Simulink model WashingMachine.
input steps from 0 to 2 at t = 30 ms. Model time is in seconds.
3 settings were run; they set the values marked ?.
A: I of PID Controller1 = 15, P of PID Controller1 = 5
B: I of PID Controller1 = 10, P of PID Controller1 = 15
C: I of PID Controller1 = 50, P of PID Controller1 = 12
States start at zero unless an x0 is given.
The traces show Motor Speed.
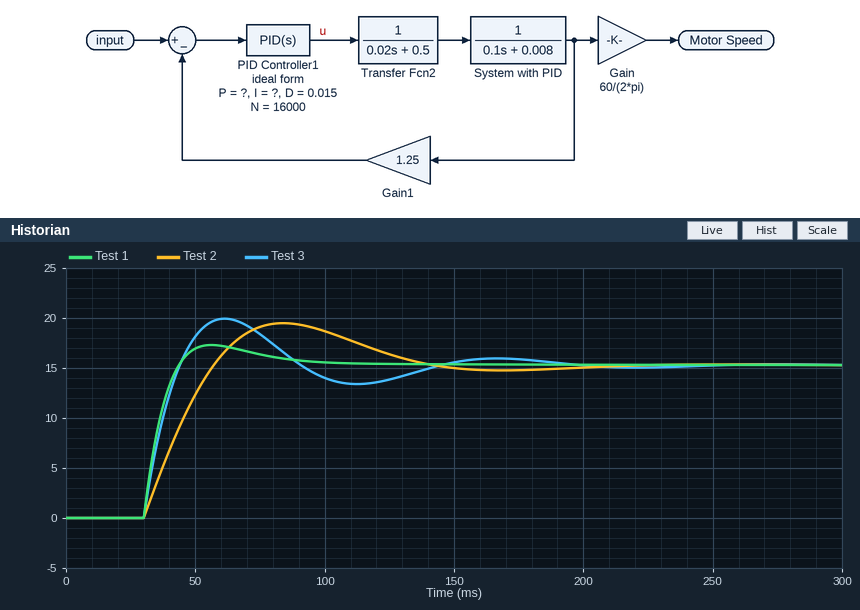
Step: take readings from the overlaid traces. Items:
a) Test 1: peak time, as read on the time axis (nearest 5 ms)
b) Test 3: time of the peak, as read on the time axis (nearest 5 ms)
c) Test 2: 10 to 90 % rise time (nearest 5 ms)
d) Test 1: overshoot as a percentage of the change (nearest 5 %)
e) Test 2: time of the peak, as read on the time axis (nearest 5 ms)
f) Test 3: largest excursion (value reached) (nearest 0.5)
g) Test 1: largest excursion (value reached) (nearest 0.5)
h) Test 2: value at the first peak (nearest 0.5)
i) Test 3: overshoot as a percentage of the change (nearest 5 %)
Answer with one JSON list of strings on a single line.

["55 ms", "60 ms", "20 ms", "15 %", "85 ms", "20.0", "17.5", "19.5", "30 %"]
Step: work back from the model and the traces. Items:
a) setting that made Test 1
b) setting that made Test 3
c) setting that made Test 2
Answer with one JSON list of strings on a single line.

["B", "C", "A"]
